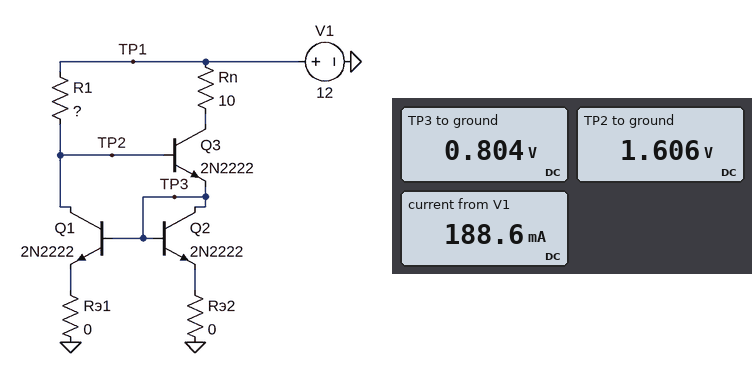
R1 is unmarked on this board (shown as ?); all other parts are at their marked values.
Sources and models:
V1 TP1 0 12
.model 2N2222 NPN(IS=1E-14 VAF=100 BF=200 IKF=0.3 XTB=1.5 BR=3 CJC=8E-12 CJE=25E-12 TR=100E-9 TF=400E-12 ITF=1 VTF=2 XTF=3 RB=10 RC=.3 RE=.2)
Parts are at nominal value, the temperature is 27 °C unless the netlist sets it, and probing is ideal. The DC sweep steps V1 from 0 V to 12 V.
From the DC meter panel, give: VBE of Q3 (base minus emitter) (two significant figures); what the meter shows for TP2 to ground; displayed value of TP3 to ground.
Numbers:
800 mV
1.606 V
0.804 V
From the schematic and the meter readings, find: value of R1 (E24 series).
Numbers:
110 Ω
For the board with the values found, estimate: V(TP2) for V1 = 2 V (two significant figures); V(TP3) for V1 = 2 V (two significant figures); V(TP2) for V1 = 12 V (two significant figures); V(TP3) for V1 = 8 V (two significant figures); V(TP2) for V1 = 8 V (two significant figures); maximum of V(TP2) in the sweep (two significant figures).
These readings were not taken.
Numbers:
1.4 V
700 mV
1.6 V
780 mV
1.6 V
1.6 V
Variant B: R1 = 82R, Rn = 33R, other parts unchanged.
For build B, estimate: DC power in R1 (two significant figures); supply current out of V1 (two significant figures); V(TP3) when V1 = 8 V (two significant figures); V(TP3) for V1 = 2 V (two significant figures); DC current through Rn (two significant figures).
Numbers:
1.3 W
250 mA
790 mV
710 mV
130 mA
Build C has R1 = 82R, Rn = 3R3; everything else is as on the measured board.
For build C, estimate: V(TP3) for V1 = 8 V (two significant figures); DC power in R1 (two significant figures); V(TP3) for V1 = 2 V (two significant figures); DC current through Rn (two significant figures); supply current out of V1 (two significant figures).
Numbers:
790 mV
1.3 W
710 mV
130 mA
250 mA
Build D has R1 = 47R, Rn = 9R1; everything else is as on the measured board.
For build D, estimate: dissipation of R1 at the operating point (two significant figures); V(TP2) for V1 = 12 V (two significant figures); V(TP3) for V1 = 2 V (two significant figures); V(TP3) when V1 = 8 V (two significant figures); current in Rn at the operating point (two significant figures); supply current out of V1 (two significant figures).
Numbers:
2.2 W
1.7 V
720 mV
830 mV
220 mA
440 mA
